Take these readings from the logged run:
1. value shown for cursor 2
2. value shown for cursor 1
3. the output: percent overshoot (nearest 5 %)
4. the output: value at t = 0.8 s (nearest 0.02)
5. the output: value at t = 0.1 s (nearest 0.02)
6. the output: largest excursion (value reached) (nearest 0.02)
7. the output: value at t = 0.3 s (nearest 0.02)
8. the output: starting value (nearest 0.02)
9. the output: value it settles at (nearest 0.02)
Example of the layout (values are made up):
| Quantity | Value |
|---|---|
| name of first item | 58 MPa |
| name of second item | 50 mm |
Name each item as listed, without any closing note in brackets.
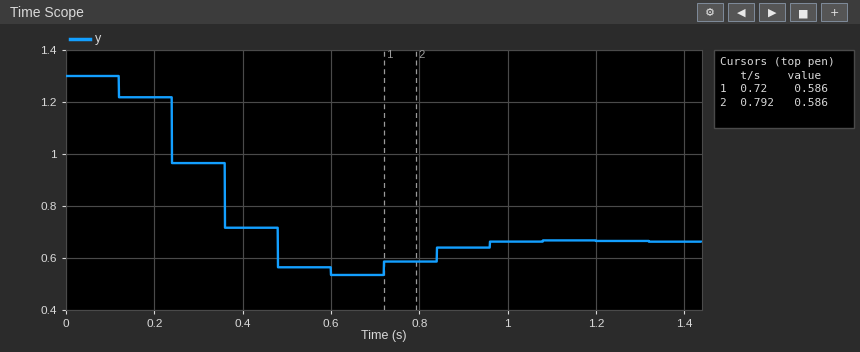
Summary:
| Quantity | Value |
|---|---|
| value shown for cursor 2 | 0.586 |
| value shown for cursor 1 | 0.586 |
| the output: percent overshoot | 20 % |
| the output: value at t = 0.8 s | 0.58 |
| the output: value at t = 0.1 s | 1.30 |
| the output: largest excursion (value reached) | 0.54 |
| the output: value at t = 0.3 s | 0.96 |
| the output: starting value | 1.30 |
| the output: value it settles at | 0.66 |
